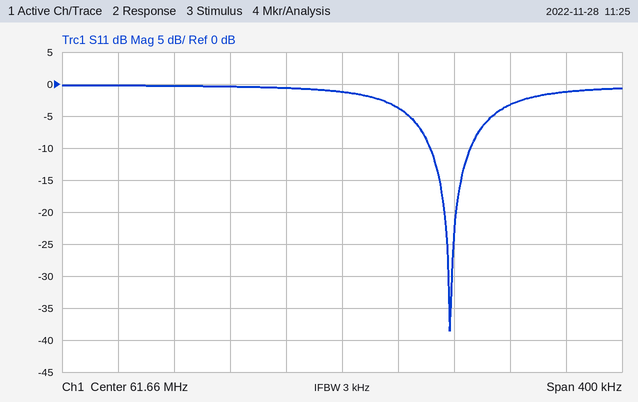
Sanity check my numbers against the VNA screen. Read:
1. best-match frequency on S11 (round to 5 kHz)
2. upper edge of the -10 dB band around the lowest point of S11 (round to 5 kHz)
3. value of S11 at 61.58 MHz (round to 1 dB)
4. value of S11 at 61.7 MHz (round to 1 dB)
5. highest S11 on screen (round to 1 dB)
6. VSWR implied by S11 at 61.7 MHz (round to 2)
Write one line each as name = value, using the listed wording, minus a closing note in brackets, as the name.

best-match frequency on S11 = 61.735 MHz
upper edge of the -10 dB band around the lowest point of S11 = 61.750 MHz
value of S11 at 61.58 MHz = 0 dB
value of S11 at 61.7 MHz = -4 dB
highest S11 on screen = 0 dB
VSWR implied by S11 at 61.7 MHz = 4
